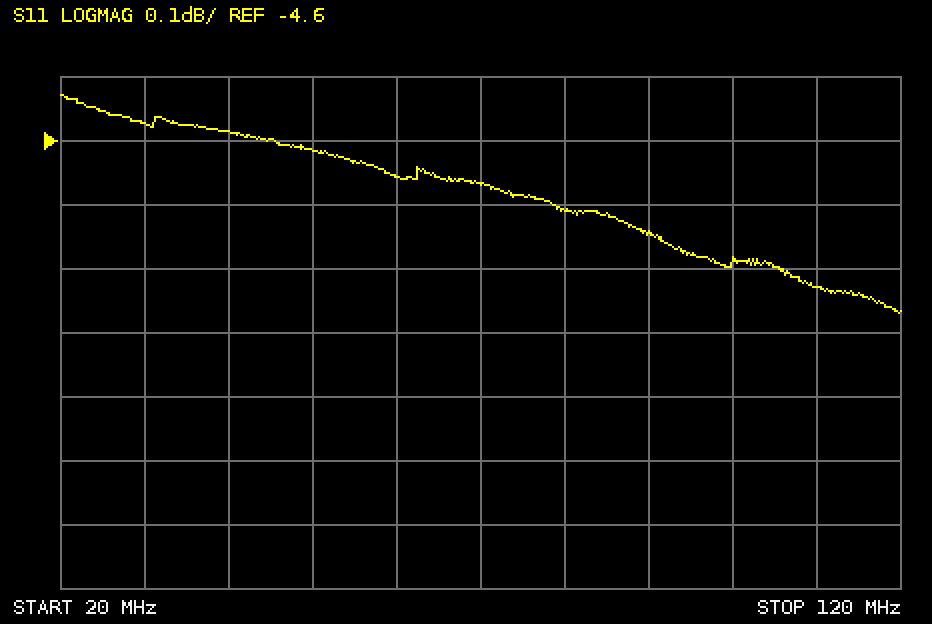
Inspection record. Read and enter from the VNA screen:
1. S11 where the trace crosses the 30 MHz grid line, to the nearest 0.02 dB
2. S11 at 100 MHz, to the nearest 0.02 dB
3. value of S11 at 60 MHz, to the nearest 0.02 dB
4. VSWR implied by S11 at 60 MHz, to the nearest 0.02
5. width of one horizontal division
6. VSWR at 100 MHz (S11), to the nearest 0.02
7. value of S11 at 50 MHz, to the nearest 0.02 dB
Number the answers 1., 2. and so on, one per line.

1. -4.58 dB
2. -4.78 dB
3. -4.66 dB
4. 3.82
5. 10 MHz
6. 3.72
7. -4.62 dB
